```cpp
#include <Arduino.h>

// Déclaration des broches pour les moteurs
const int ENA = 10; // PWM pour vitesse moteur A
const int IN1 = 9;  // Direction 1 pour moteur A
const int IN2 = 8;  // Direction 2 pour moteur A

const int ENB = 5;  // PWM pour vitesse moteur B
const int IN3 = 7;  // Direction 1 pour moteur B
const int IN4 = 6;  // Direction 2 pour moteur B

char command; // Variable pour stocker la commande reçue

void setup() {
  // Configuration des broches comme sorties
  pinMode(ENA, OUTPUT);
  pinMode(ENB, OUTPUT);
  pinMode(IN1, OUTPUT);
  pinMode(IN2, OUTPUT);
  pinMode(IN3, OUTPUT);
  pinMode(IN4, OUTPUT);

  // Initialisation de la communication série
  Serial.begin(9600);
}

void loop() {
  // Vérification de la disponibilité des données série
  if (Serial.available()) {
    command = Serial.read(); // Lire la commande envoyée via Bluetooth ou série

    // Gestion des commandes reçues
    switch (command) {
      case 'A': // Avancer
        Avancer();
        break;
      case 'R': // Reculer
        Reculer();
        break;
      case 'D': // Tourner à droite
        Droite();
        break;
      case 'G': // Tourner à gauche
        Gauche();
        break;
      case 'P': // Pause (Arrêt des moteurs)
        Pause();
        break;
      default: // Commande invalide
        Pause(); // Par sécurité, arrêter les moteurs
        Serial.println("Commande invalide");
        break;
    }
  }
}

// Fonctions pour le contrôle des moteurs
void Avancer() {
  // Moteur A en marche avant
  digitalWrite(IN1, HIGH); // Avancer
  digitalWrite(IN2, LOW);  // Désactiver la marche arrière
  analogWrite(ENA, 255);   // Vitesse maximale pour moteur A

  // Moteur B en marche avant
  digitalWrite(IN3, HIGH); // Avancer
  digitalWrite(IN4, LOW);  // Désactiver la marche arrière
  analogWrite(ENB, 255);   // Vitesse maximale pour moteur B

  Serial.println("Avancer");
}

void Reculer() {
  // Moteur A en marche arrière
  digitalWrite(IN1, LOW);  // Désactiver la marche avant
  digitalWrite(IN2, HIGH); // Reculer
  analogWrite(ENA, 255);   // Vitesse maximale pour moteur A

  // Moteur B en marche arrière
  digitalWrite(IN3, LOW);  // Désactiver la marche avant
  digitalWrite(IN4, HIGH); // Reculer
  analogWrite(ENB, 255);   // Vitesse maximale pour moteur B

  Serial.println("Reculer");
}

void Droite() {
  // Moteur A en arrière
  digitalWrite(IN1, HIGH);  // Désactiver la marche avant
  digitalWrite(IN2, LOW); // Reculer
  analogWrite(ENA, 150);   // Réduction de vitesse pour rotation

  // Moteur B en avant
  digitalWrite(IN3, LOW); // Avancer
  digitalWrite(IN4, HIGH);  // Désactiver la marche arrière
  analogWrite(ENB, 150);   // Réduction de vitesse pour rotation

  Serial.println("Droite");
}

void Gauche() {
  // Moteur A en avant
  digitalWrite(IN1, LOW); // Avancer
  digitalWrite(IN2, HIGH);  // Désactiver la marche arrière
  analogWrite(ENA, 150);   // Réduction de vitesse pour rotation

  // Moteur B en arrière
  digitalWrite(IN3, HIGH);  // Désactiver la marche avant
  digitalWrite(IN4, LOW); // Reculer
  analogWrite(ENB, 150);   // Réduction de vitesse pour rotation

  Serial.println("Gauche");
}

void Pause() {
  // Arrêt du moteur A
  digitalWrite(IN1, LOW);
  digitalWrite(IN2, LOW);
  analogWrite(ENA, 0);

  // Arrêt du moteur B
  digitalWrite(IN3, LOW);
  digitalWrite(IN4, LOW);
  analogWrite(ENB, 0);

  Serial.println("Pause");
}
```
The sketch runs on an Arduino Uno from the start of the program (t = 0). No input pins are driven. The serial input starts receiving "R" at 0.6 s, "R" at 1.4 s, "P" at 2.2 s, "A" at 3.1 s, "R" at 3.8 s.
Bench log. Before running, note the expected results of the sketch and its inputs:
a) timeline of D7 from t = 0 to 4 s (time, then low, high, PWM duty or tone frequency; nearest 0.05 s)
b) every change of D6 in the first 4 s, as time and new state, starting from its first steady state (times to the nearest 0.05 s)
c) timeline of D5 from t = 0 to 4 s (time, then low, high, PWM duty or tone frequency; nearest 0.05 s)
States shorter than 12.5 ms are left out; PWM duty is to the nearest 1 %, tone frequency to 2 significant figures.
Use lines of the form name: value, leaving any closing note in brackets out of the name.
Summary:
timeline of D7 from t = 0 to 4 s: 0 s low; 3.1 s high; 3.8 s low
every change of D6 in the first 4 s, as time and new state, starting from its first steady state: 0 s low; 0.6 s high; 2.2 s low; 3.8 s high
timeline of D5 from t = 0 to 4 s: 0 s low; 0.6 s high; 2.2 s low; 3.1 s high
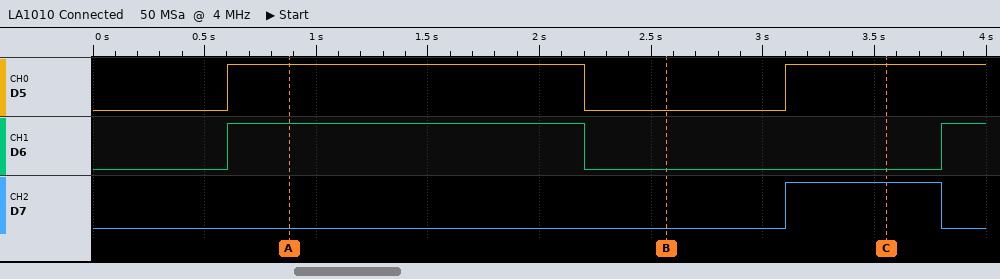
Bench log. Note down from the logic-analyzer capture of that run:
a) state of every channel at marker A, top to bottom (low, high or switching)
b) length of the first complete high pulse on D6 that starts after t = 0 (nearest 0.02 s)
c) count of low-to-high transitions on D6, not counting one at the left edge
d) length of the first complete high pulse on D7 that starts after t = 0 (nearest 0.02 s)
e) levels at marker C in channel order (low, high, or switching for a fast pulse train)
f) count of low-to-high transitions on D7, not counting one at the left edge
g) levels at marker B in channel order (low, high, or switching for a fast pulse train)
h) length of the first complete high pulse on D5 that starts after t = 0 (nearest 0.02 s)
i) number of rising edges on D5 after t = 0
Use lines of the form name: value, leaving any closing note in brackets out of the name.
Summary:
state of every channel at marker A, top to bottom: D5 high, D6 high, D7 low
length of the first complete high pulse on D6 that starts after t = 0: 1.60 s
count of low-to-high transitions on D6, not counting one at the left edge: 2
length of the first complete high pulse on D7 that starts after t = 0: 0.70 s
levels at marker C in channel order: D5 high, D6 low, D7 high
count of low-to-high transitions on D7, not counting one at the left edge: 1
levels at marker B in channel order: D5 low, D6 low, D7 low
length of the first complete high pulse on D5 that starts after t = 0: 1.60 s
number of rising edges on D5 after t = 0: 2
